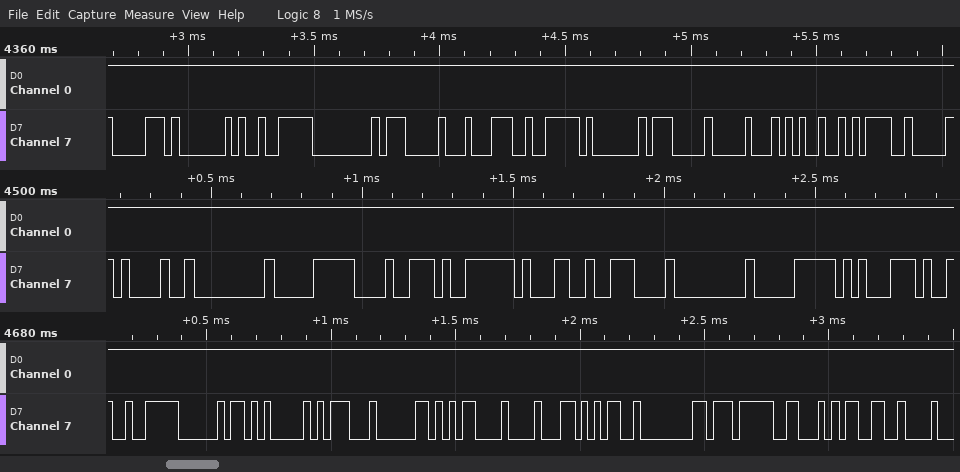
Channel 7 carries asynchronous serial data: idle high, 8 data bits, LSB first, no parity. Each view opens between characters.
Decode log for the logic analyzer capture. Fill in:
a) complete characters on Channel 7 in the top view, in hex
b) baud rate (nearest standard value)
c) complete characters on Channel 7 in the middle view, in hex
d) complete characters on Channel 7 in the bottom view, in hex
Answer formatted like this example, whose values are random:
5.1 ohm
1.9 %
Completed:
70, 40, F2, 00, 07, C4, F2, 01, 07, 10, 25, 3D
38400 baud
21, 00, F0, C8, F9, 31, 0E, 00, F0, C5
F2, A0, 05, 1D, 60, 0D, 88, 35, 80, F7, 46, 33
